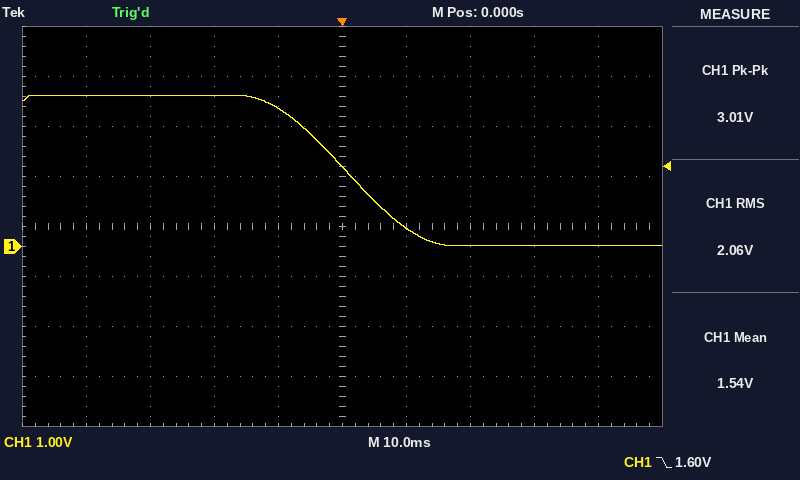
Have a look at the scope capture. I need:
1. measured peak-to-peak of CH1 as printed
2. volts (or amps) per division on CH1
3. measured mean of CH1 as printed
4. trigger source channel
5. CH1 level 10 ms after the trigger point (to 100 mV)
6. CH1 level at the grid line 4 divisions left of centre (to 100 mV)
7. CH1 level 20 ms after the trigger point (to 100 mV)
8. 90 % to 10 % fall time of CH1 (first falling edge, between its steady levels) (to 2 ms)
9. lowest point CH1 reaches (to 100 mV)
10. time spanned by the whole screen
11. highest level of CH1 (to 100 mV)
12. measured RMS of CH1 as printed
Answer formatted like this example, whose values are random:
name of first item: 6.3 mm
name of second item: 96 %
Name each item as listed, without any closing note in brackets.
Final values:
measured peak-to-peak of CH1 as printed: 3.01 V
volts (or amps) per division on CH1: 1 V
measured mean of CH1 as printed: 1.54 V
trigger source channel: CH1
CH1 level 10 ms after the trigger point: 400 mV
CH1 level at the grid line 4 divisions left of centre: 3.0 V
CH1 level 20 ms after the trigger point: 0.0 V
90 % to 10 % fall time of CH1 (first falling edge, between its steady levels): 20 ms
lowest point CH1 reaches: 0.0 V
time spanned by the whole screen: 100 ms
highest level of CH1: 3.0 V
measured RMS of CH1 as printed: 2.06 V
